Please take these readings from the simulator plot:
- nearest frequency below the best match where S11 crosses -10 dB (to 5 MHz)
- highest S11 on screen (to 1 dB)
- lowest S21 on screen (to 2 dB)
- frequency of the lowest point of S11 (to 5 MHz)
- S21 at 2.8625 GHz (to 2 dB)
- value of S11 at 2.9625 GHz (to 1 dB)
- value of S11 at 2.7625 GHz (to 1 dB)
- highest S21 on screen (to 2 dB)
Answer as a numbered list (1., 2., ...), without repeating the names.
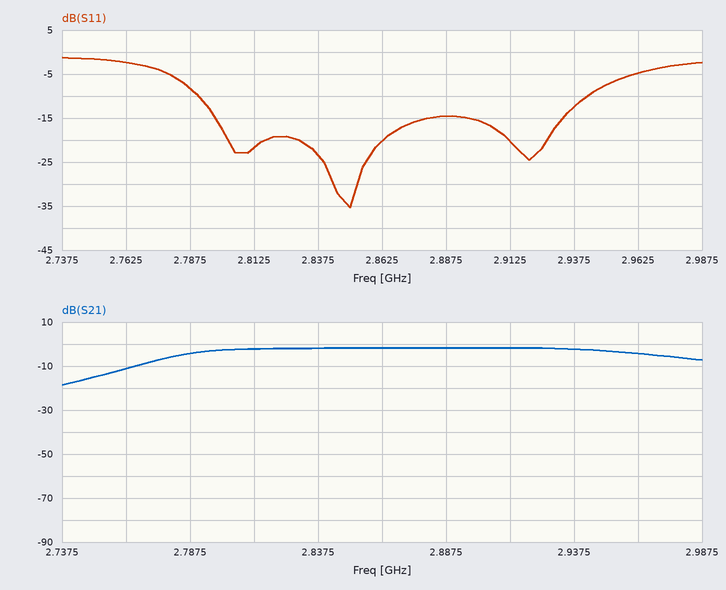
1. 2.790 GHz
2. -1 dB
3. -18 dB
4. 2.850 GHz
5. -2 dB
6. -5 dB
7. -2 dB
8. -2 dB
